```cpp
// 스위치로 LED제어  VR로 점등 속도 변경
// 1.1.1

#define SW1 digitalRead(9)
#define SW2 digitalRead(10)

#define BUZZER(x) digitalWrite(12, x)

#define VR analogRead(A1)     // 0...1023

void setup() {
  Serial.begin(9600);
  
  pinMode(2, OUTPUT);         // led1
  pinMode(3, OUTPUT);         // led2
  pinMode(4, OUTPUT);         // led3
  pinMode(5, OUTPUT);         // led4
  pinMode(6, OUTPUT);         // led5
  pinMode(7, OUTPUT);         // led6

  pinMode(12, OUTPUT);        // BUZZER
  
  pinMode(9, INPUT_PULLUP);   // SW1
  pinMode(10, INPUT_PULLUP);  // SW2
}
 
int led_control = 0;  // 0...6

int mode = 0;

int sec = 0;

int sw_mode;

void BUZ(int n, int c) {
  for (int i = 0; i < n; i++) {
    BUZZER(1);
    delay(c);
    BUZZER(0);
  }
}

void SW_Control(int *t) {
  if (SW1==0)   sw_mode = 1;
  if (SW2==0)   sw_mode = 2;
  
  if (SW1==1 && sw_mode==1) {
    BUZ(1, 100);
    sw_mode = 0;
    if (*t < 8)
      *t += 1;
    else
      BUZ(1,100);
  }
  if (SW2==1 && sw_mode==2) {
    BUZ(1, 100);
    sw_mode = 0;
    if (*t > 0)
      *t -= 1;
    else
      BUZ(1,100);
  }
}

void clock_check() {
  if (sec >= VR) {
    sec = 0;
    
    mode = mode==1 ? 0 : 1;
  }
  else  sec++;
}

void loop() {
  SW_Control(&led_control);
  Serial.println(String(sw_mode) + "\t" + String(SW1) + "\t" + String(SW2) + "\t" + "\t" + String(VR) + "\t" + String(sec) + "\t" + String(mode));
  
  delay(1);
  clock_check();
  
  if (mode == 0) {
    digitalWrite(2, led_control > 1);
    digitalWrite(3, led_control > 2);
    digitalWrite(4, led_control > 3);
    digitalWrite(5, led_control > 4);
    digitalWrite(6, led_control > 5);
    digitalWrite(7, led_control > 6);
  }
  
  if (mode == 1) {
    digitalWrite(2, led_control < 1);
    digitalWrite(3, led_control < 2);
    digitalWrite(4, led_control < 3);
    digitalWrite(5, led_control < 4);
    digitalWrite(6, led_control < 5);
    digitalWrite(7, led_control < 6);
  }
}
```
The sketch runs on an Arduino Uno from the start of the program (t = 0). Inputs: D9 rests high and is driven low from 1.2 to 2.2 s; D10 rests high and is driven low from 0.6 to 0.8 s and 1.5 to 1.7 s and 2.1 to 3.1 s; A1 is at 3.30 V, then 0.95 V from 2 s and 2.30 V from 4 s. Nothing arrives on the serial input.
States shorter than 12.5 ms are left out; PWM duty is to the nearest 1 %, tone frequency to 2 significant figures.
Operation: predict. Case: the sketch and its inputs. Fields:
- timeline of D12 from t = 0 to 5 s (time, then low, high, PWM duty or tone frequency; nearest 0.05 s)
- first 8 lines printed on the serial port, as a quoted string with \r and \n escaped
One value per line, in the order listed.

0 s low; 0.8 s high; 1 s low; 3.1 s high; 3.3 s low
"0\t1\t1\t\t675\t0\t0\r\n0\t1\t1\t\t675\t1\t0\r\n0\t1\t1\t\t675\t2\t0\r\n0\t1\t1\t\t675\t3\t0\r\n0\t1\t1\t\t675\t4\t0\r\n0\t1\t1\t\t675\t5\t0\r\n0\t1\t1\t\t675\t6\t0\r\n0\t1\t1\t\t675\t7\t0\r\n"
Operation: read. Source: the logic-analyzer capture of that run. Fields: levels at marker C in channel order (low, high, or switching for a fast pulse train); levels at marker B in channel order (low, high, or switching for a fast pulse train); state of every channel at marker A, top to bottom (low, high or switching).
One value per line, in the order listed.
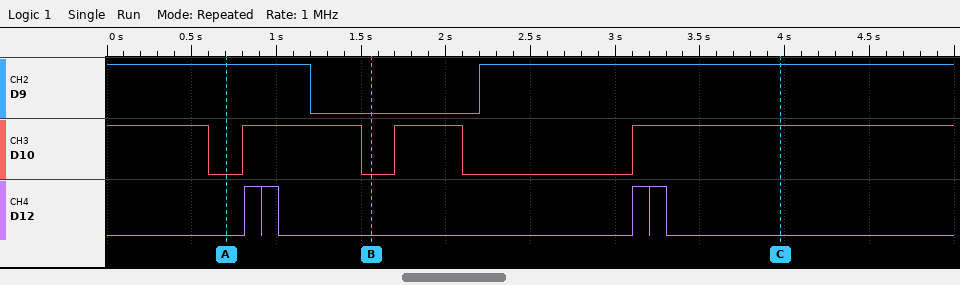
D9 high, D10 high, D12 low
D9 low, D10 low, D12 low
D9 high, D10 low, D12 low
